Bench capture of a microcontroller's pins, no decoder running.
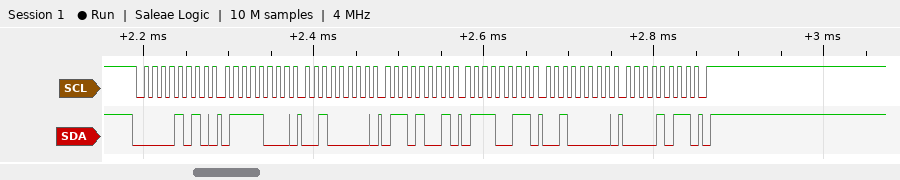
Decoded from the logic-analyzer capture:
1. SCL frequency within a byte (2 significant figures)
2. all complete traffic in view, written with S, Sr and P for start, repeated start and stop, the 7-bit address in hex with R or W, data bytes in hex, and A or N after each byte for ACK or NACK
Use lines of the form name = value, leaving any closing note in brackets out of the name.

SCL frequency within a byte = 100 kHz
all complete traffic in view, written with S, Sr and P for start, repeated start and stop, the 7-bit address in hex with R or W, data bytes in hex, and A or N after each byte for ACK or NACK = S 05W A 78 A 20 A 69 A 73 A 20 A 0B A P
